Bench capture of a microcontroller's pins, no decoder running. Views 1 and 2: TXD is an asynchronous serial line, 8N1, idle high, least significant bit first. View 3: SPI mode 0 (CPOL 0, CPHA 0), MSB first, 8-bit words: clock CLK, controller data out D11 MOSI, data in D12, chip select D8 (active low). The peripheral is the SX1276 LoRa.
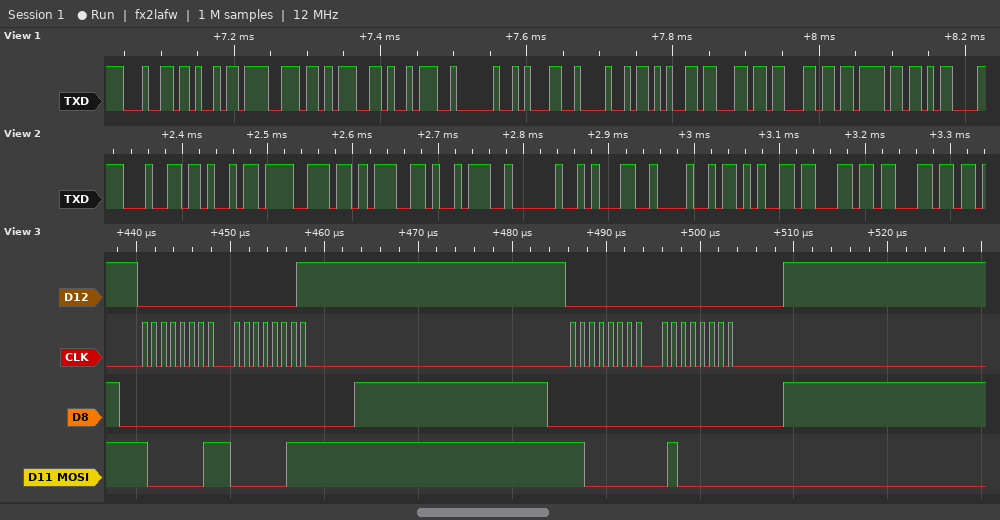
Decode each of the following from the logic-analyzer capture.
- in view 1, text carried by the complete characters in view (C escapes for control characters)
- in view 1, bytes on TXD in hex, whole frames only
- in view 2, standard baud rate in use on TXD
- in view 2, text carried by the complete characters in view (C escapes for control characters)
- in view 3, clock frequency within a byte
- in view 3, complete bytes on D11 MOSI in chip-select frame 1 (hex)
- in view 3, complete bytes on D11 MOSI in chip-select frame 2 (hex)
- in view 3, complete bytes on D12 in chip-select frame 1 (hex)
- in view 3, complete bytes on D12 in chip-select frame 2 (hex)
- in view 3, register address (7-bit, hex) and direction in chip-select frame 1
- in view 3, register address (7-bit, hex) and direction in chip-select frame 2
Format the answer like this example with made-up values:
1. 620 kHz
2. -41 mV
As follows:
1. "ding: 1Hello\r"
2. 0x64 0x69 0x6E 0x67 0x3A 0x20 0x31 0x48 0x65 0x6C 0x6C 0x6F 0x0D
3. 115200 baud
4. "ding: 1Hell"
5. 1 MHz
6. 81 03
7. C0 40
8. 00 01
9. 00 00
10. 0x01 write
11. 0x40 write
